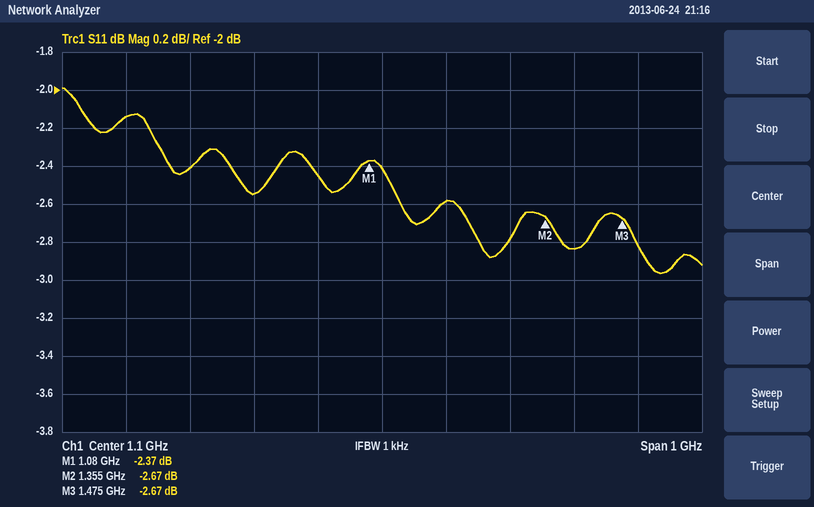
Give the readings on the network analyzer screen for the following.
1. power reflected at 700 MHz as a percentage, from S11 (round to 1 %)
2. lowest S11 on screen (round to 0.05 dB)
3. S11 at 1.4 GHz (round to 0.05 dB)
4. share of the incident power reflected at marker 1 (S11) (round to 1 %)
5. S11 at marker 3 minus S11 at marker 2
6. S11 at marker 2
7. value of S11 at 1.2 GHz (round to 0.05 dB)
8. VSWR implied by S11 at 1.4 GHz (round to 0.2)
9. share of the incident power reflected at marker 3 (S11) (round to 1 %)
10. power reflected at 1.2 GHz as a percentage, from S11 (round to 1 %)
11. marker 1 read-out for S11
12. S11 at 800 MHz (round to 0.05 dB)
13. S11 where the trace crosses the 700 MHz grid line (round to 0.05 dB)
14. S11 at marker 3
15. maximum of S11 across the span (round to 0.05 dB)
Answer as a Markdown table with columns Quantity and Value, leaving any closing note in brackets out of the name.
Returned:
| Quantity | Value |
|---|---|
| power reflected at 700 MHz as a percentage, from S11 | 61 % |
| lowest S11 on screen | -2.95 dB |
| S11 at 1.4 GHz | -2.85 dB |
| share of the incident power reflected at marker 1 (S11) | 58 % |
| S11 at marker 3 minus S11 at marker 2 | 0.00 dB |
| S11 at marker 2 | -2.67 dB |
| value of S11 at 1.2 GHz | -2.60 dB |
| VSWR implied by S11 at 1.4 GHz | 6.2 |
| share of the incident power reflected at marker 3 (S11) | 54 % |
| power reflected at 1.2 GHz as a percentage, from S11 | 55 % |
| marker 1 read-out for S11 | -2.37 dB |
| S11 at 800 MHz | -2.40 dB |
| S11 where the trace crosses the 700 MHz grid line | -2.15 dB |
| S11 at marker 3 | -2.67 dB |
| maximum of S11 across the span | -2.00 dB |
